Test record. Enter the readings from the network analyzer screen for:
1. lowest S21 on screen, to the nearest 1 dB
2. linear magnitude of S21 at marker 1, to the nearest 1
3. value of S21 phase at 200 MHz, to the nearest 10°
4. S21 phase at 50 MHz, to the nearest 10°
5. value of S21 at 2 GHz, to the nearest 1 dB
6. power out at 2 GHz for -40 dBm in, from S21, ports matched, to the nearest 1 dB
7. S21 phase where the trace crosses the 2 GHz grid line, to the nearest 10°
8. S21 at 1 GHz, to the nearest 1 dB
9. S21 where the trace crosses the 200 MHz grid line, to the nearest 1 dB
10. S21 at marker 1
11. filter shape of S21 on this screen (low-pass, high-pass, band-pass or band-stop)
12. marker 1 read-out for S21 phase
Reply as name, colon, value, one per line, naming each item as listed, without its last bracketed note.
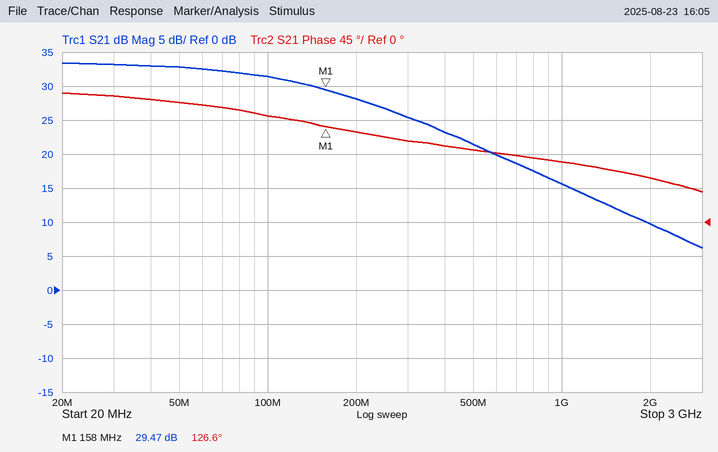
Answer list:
lowest S21 on screen, to the nearest 1 dB: 6 dB
linear magnitude of S21 at marker 1, to the nearest 1: 30
value of S21 phase at 200 MHz, to the nearest 10°: 120°
S21 phase at 50 MHz, to the nearest 10°: 160°
value of S21 at 2 GHz, to the nearest 1 dB: 10 dB
power out at 2 GHz for -40 dBm in, from S21, ports matched, to the nearest 1 dB: -30 dBm
S21 phase where the trace crosses the 2 GHz grid line, to the nearest 10°: 60°
S21 at 1 GHz, to the nearest 1 dB: 16 dB
S21 where the trace crosses the 200 MHz grid line, to the nearest 1 dB: 28 dB
S21 at marker 1: 29.47 dB
filter shape of S21 on this screen: low-pass
marker 1 read-out for S21 phase: 126.6°
